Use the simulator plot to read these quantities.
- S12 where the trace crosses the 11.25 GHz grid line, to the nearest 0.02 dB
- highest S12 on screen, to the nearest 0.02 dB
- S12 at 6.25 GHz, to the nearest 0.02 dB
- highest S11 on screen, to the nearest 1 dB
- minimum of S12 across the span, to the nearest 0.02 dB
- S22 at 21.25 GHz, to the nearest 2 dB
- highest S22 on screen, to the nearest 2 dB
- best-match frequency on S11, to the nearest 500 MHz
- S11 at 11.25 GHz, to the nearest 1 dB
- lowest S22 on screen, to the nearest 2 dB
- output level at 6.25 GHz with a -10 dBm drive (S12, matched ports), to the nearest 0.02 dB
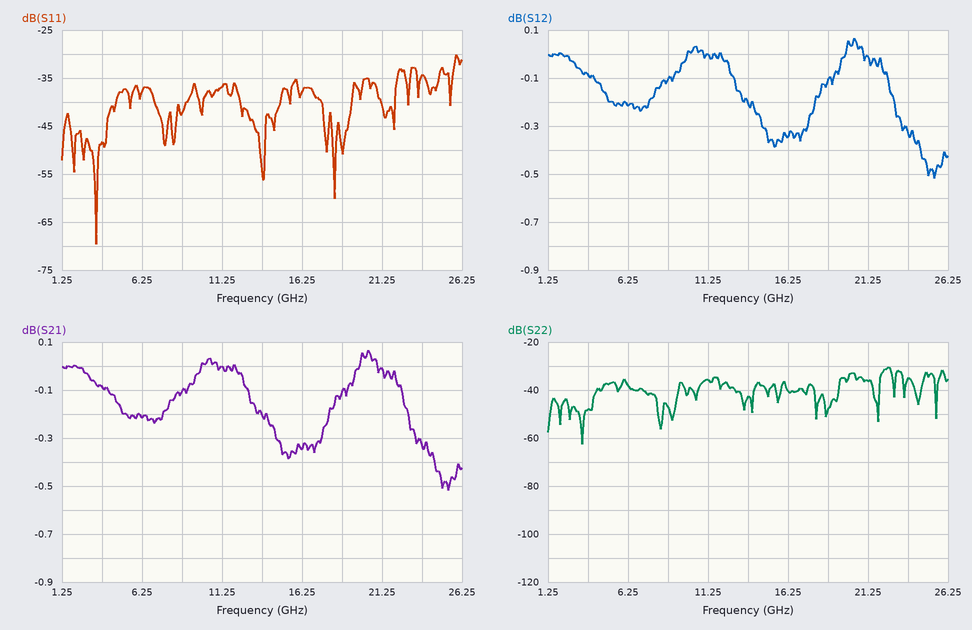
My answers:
0.00 dB
0.06 dB
-0.22 dB
-30 dB
-0.52 dB
-36 dB
-30 dB
3.5 GHz
-37 dB
-62 dB
-10.22 dBm
